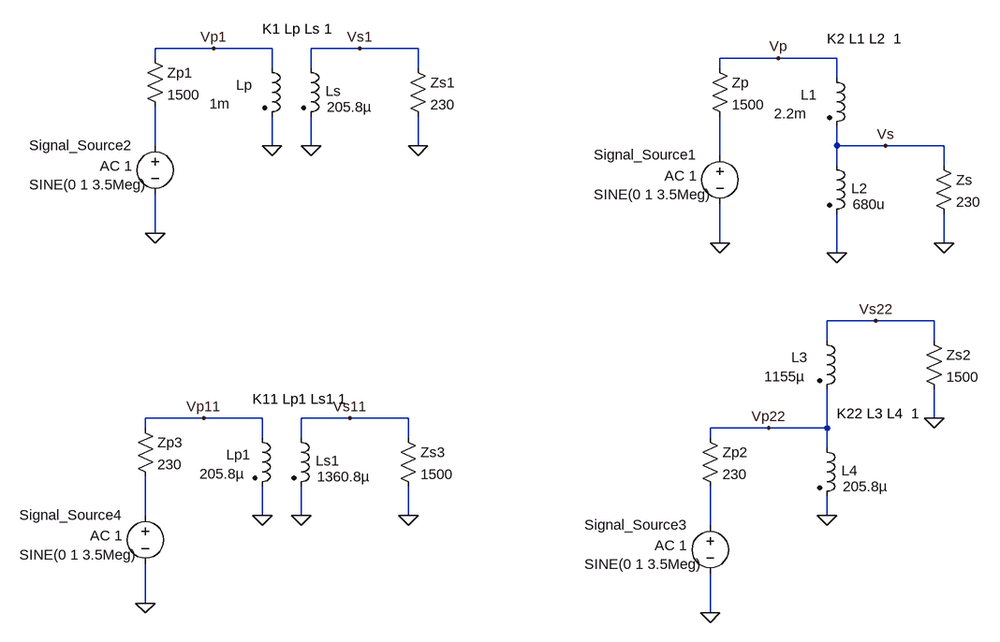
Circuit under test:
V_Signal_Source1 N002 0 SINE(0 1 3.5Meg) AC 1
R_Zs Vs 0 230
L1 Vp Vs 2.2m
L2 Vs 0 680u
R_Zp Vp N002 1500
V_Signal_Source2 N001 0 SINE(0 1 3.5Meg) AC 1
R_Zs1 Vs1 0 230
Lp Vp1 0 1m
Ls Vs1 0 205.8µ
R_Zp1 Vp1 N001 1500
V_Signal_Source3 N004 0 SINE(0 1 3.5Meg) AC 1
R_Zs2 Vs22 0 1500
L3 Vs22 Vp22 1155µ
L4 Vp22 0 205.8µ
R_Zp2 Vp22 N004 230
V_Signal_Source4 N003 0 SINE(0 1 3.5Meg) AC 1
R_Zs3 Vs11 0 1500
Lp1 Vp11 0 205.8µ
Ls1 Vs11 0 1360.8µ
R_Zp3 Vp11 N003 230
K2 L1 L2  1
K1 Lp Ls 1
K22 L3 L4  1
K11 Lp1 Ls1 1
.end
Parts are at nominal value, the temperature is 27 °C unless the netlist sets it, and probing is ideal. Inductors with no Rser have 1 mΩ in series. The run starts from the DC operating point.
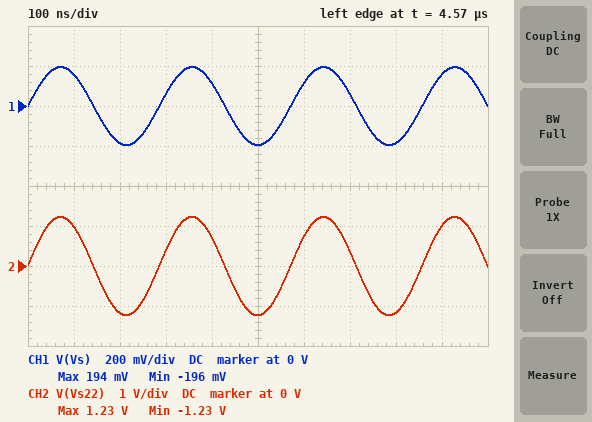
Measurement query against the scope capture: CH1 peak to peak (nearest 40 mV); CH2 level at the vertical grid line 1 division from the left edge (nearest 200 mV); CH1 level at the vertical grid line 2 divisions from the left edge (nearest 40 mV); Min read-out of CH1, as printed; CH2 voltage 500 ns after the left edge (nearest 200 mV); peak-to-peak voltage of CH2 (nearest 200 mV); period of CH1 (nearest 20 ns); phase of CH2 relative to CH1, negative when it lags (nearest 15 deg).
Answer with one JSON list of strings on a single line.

["400 mV", "1.0 V", "-200 mV", "-196 mV", "-1.2 V", "2.4 V", "280 ns", "0 deg"]
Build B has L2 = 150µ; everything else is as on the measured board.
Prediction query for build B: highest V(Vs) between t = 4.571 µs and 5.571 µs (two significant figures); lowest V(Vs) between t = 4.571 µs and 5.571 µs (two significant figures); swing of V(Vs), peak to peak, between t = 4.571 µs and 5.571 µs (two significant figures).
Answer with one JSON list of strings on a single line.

["160 mV", "-160 mV", "320 mV"]
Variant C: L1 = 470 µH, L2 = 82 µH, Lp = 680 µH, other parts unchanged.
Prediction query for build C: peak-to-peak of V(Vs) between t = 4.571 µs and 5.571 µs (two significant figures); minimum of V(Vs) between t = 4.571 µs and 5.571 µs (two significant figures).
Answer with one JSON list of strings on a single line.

["380 mV", "-190 mV"]
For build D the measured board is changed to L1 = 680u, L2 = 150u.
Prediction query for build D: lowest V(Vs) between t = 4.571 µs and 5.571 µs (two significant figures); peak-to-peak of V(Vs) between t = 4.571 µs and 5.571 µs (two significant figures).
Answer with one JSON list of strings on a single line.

["-190 mV", "380 mV"]
